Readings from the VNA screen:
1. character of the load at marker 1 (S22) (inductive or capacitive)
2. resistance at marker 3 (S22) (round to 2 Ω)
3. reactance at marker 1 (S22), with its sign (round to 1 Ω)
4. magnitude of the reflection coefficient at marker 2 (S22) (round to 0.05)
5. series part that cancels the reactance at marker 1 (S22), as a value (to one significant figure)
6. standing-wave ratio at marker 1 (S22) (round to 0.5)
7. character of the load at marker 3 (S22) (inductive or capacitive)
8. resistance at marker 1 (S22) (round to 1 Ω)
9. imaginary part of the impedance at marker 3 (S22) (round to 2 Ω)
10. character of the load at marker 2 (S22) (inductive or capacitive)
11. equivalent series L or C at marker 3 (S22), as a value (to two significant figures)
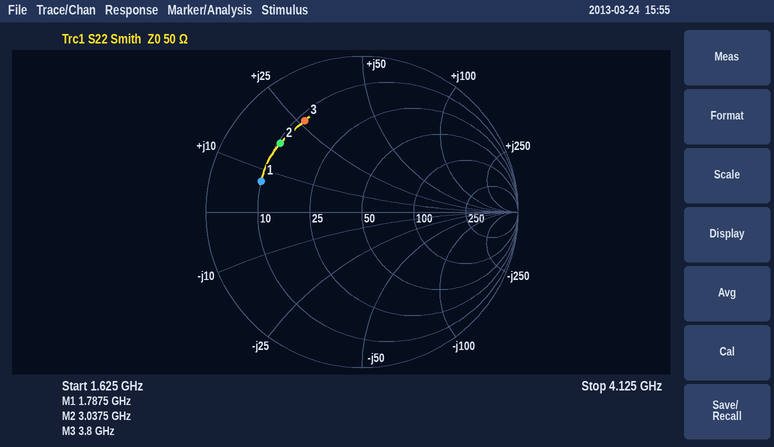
inductive
12 Ω
+7 Ω
0.70
10 pF
5.0
inductive
10 Ω
+26 Ω
inductive
1.1 nH
